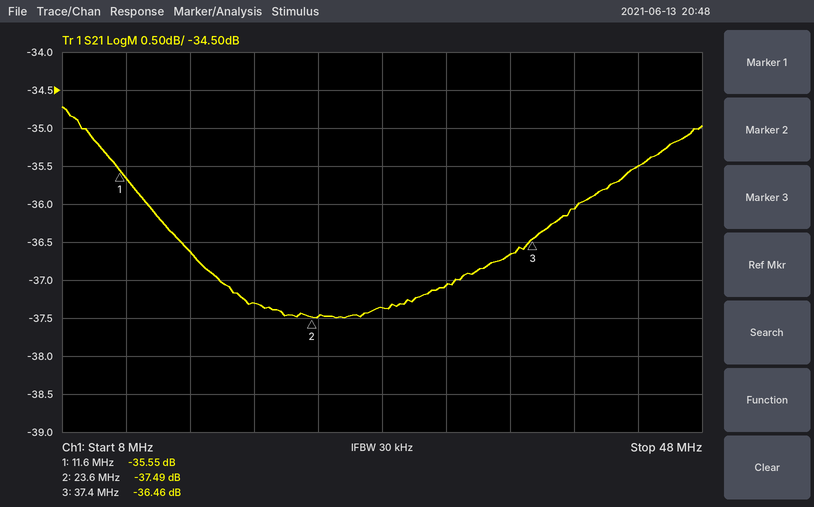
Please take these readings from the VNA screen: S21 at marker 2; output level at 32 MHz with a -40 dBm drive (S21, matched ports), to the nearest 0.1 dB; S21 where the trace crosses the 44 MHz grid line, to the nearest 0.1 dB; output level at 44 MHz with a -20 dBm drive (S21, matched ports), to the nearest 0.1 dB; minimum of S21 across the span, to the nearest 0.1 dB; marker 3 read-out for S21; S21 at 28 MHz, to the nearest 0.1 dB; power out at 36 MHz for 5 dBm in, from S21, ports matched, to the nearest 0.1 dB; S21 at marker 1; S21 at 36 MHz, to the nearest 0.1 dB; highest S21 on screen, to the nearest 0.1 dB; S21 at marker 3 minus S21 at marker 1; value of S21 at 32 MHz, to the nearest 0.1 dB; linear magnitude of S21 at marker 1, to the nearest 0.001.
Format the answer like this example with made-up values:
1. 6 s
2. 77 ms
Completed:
1. -37.49 dB
2. -77.1 dBm
3. -35.5 dB
4. -55.5 dBm
5. -37.5 dB
6. -36.46 dB
7. -37.4 dB
8. -31.7 dBm
9. -35.55 dB
10. -36.7 dB
11. -34.7 dB
12. -0.91 dB
13. -37.1 dB
14. 0.017
